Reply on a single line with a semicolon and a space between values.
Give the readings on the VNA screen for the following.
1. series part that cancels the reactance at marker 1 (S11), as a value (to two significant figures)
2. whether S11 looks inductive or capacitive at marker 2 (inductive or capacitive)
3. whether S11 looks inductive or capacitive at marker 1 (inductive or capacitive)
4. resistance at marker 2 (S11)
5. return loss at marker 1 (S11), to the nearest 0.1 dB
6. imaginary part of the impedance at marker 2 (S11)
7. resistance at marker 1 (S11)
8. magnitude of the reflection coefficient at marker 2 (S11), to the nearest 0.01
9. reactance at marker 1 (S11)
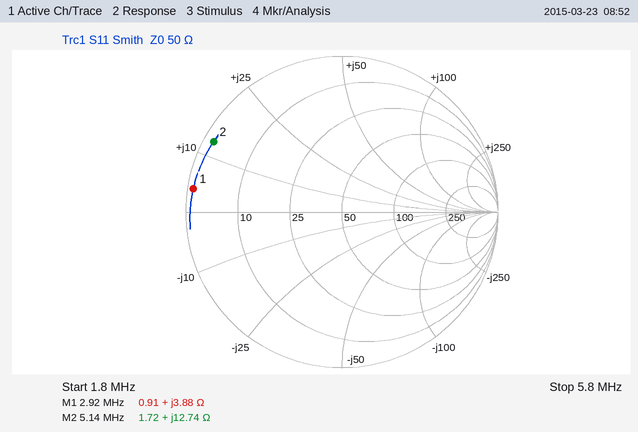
14 nF; inductive; inductive; 1.72 Ω; 0.3 dB; +12.74 Ω; 0.91 Ω; 0.94; +3.88 Ω
